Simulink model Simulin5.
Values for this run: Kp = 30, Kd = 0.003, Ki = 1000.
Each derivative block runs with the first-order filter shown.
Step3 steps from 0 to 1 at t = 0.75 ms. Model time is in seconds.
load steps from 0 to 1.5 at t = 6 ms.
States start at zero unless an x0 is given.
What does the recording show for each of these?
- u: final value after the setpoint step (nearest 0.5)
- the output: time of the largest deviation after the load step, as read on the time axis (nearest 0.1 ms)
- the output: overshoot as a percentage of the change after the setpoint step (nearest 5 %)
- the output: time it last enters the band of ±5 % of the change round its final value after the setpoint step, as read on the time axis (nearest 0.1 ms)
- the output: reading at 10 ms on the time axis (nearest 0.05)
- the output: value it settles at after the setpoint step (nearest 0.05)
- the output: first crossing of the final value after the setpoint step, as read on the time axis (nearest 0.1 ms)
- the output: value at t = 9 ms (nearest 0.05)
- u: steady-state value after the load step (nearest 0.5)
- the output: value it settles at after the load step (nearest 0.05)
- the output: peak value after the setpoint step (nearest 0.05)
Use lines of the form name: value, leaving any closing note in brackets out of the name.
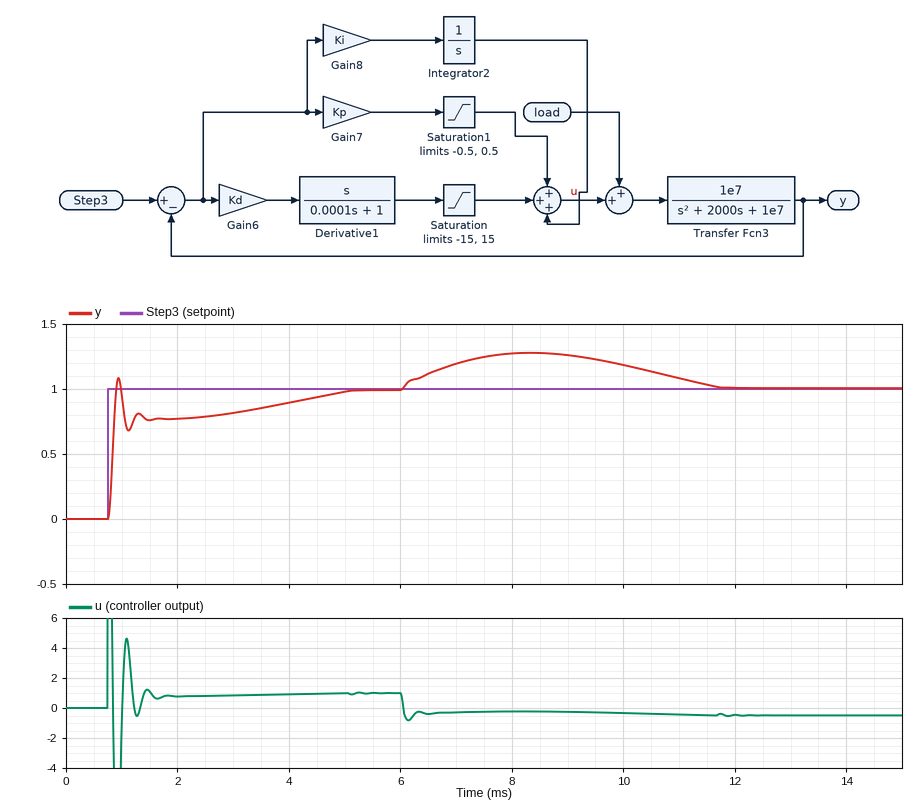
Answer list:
u: final value after the setpoint step: 1.0
the output: time of the largest deviation after the load step, as read on the time axis: 8.3 ms
the output: overshoot as a percentage of the change after the setpoint step: 10 %
the output: time it last enters the band of ±5 % of the change round its final value after the setpoint step, as read on the time axis: 4.6 ms
the output: reading at 10 ms on the time axis: 1.20
the output: value it settles at after the setpoint step: 1.00
the output: first crossing of the final value after the setpoint step, as read on the time axis: 0.9 ms
the output: value at t = 9 ms: 1.25
u: steady-state value after the load step: -0.5
the output: value it settles at after the load step: 1.00
the output: peak value after the setpoint step: 1.10
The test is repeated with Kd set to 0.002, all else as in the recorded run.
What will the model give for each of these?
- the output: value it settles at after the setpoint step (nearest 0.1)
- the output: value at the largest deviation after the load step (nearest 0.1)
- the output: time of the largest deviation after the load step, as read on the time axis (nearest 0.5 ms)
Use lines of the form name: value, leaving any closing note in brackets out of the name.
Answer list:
the output: value it settles at after the setpoint step: 1.0
the output: value at the largest deviation after the load step: 1.3
the output: time of the largest deviation after the load step, as read on the time axis: 8.0 ms
